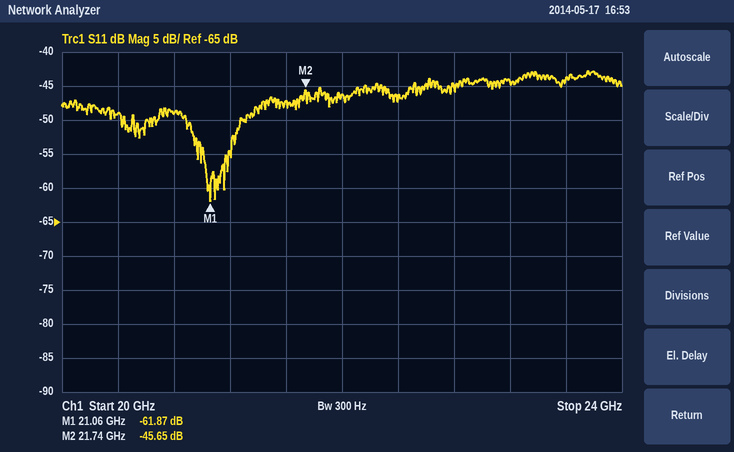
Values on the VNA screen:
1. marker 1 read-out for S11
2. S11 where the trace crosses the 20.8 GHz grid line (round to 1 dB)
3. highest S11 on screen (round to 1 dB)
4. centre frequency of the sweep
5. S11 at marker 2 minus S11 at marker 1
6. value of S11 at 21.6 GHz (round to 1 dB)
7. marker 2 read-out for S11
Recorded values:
-61.87 dB
-49 dB
-43 dB
22 GHz
16.22 dB
-47 dB
-45.65 dB
